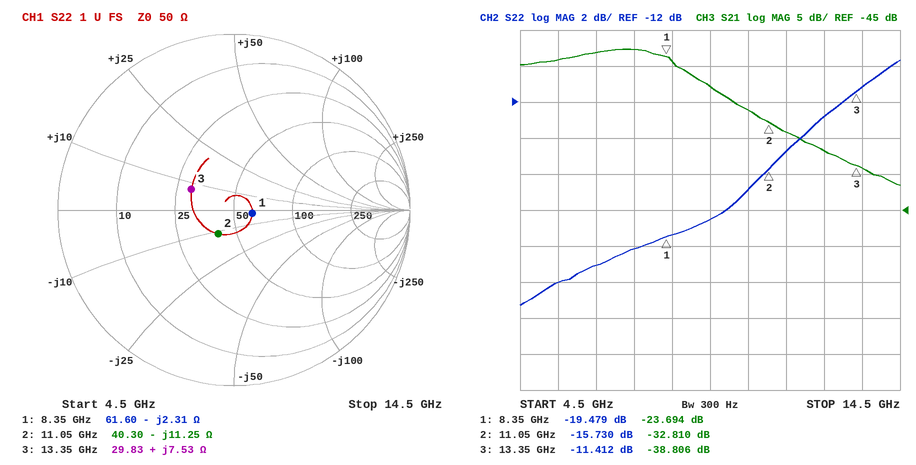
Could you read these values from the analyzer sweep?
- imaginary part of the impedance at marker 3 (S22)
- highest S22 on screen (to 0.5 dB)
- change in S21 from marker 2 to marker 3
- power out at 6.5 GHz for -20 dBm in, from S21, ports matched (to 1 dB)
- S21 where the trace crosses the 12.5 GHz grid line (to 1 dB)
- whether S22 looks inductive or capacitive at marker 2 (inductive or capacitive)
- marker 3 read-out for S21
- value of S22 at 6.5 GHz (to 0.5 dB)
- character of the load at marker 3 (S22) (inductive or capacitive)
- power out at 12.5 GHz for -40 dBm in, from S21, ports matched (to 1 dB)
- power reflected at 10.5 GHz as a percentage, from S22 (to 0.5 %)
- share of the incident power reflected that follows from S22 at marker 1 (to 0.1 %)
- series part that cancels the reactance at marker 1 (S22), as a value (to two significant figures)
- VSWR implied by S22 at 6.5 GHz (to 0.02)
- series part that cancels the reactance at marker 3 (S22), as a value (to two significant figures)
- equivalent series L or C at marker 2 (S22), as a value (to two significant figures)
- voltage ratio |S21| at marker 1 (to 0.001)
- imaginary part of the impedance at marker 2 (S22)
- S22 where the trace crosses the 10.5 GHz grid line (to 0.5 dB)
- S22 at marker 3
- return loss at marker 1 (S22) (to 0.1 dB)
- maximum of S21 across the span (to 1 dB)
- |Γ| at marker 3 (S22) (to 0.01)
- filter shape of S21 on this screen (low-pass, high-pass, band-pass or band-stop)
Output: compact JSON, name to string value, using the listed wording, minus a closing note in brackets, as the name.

{"imaginary part of the impedance at marker 3": "+7.53 Ω", "highest S22 on screen": "-9.5 dB", "change in S21 from marker 2 to marker 3": "-5.996 dB", "power out at 6.5 GHz for -20 dBm in, from S21, ports matched": "-43 dBm", "S21 where the trace crosses the 12.5 GHz grid line": "-37 dB", "whether S22 looks inductive or capacitive at marker 2": "capacitive", "marker 3 read-out for S21": "-38.806 dB", "value of S22 at 6.5 GHz": "-21.0 dB", "character of the load at marker 3 (S22)": "inductive", "power out at 12.5 GHz for -40 dBm in, from S21, ports matched": "-77 dBm", "power reflected at 10.5 GHz as a percentage, from S22": "2.0 %", "share of the incident power reflected that follows from S22 at marker 1": "1.1 %", "series part that cancels the reactance at marker 1 (S22), as a value": "44 pH", "VSWR implied by S22 at 6.5 GHz": "1.20", "series part that cancels the reactance at marker 3 (S22), as a value": "1.6 pF", "equivalent series L or C at marker 2 (S22), as a value": "1.3 pF", "voltage ratio |S21| at marker 1": "0.065", "imaginary part of the impedance at marker 2": "-11.25 Ω", "S22 where the trace crosses the 10.5 GHz grid line": "-17.0 dB", "S22 at marker 3": "-11.412 dB", "return loss at marker 1 (S22)": "19.5 dB", "maximum of S21 across the span": "-23 dB", "|Γ| at marker 3 (S22)": "0.27", "filter shape of S21 on this screen": "low-pass"}
